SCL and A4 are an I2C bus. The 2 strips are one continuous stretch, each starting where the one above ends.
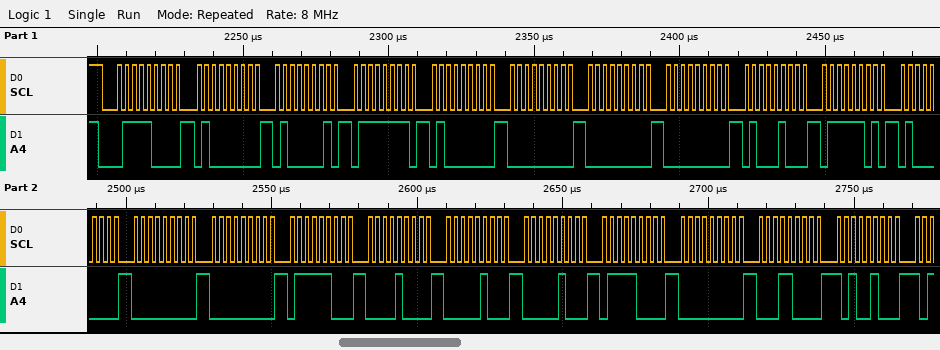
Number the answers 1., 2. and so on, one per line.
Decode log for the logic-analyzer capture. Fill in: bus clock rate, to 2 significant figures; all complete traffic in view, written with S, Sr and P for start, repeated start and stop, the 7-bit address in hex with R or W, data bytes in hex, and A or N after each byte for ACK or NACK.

1. 400 kHz
2. S 3CW A 40 A 41 A 7F A 40 A 00 A 00 A 00 A 44 A 7D A 40 A 00 A 00 A 7C A 08 A 04 A 04 A 78 A 00 A 18 A A4 A
